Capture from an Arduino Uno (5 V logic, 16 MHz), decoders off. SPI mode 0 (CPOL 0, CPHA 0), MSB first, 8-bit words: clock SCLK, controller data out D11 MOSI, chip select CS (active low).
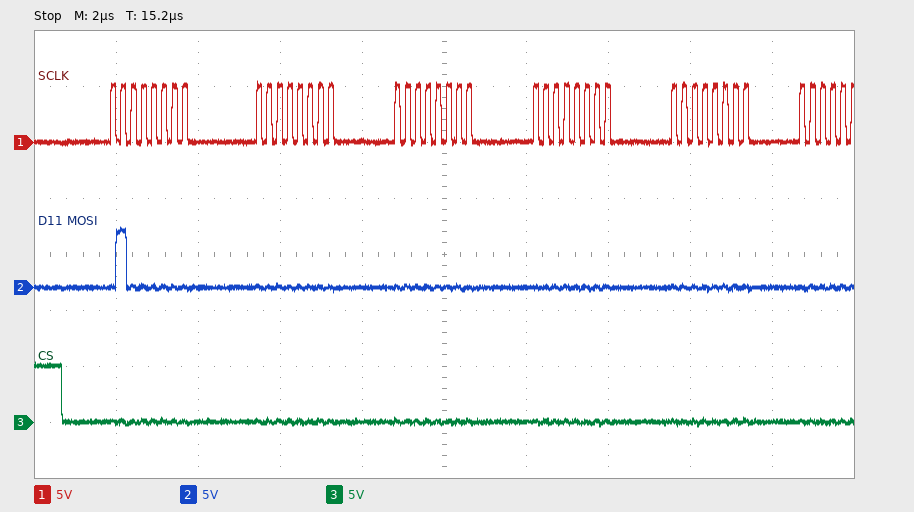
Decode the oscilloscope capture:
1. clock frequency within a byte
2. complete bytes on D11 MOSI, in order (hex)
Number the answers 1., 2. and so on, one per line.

1. 4 MHz
2. 40 00 00 00 00
